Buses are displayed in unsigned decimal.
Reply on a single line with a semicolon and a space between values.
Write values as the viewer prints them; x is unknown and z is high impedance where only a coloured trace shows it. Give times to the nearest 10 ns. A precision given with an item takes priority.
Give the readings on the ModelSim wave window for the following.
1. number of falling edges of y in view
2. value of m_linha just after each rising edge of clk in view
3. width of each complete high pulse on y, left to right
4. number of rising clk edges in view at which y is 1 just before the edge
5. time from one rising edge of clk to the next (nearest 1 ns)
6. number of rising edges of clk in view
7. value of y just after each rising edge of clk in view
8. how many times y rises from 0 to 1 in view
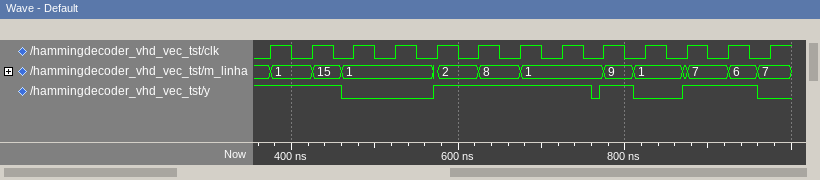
4; 1, 15, 1, 1, 2, 8, 1, 1, 9, 1, 7, 6, 7; 190 ns, 40 ns, 90 ns; 9; 50 ns; 13; 1 1 0 0 1 1 1 1 1 0 1 1 0; 3
